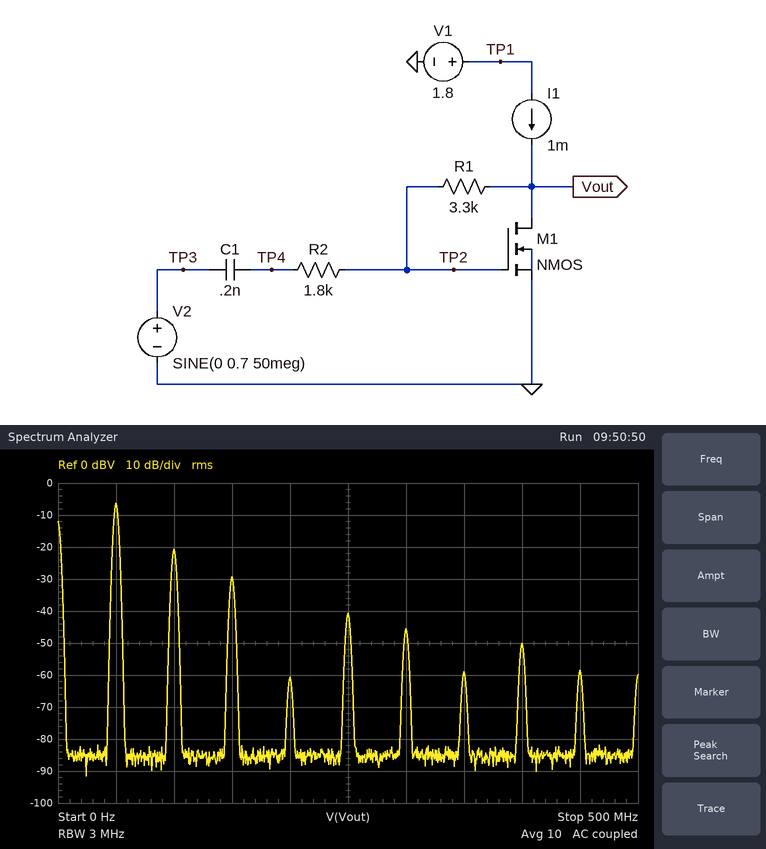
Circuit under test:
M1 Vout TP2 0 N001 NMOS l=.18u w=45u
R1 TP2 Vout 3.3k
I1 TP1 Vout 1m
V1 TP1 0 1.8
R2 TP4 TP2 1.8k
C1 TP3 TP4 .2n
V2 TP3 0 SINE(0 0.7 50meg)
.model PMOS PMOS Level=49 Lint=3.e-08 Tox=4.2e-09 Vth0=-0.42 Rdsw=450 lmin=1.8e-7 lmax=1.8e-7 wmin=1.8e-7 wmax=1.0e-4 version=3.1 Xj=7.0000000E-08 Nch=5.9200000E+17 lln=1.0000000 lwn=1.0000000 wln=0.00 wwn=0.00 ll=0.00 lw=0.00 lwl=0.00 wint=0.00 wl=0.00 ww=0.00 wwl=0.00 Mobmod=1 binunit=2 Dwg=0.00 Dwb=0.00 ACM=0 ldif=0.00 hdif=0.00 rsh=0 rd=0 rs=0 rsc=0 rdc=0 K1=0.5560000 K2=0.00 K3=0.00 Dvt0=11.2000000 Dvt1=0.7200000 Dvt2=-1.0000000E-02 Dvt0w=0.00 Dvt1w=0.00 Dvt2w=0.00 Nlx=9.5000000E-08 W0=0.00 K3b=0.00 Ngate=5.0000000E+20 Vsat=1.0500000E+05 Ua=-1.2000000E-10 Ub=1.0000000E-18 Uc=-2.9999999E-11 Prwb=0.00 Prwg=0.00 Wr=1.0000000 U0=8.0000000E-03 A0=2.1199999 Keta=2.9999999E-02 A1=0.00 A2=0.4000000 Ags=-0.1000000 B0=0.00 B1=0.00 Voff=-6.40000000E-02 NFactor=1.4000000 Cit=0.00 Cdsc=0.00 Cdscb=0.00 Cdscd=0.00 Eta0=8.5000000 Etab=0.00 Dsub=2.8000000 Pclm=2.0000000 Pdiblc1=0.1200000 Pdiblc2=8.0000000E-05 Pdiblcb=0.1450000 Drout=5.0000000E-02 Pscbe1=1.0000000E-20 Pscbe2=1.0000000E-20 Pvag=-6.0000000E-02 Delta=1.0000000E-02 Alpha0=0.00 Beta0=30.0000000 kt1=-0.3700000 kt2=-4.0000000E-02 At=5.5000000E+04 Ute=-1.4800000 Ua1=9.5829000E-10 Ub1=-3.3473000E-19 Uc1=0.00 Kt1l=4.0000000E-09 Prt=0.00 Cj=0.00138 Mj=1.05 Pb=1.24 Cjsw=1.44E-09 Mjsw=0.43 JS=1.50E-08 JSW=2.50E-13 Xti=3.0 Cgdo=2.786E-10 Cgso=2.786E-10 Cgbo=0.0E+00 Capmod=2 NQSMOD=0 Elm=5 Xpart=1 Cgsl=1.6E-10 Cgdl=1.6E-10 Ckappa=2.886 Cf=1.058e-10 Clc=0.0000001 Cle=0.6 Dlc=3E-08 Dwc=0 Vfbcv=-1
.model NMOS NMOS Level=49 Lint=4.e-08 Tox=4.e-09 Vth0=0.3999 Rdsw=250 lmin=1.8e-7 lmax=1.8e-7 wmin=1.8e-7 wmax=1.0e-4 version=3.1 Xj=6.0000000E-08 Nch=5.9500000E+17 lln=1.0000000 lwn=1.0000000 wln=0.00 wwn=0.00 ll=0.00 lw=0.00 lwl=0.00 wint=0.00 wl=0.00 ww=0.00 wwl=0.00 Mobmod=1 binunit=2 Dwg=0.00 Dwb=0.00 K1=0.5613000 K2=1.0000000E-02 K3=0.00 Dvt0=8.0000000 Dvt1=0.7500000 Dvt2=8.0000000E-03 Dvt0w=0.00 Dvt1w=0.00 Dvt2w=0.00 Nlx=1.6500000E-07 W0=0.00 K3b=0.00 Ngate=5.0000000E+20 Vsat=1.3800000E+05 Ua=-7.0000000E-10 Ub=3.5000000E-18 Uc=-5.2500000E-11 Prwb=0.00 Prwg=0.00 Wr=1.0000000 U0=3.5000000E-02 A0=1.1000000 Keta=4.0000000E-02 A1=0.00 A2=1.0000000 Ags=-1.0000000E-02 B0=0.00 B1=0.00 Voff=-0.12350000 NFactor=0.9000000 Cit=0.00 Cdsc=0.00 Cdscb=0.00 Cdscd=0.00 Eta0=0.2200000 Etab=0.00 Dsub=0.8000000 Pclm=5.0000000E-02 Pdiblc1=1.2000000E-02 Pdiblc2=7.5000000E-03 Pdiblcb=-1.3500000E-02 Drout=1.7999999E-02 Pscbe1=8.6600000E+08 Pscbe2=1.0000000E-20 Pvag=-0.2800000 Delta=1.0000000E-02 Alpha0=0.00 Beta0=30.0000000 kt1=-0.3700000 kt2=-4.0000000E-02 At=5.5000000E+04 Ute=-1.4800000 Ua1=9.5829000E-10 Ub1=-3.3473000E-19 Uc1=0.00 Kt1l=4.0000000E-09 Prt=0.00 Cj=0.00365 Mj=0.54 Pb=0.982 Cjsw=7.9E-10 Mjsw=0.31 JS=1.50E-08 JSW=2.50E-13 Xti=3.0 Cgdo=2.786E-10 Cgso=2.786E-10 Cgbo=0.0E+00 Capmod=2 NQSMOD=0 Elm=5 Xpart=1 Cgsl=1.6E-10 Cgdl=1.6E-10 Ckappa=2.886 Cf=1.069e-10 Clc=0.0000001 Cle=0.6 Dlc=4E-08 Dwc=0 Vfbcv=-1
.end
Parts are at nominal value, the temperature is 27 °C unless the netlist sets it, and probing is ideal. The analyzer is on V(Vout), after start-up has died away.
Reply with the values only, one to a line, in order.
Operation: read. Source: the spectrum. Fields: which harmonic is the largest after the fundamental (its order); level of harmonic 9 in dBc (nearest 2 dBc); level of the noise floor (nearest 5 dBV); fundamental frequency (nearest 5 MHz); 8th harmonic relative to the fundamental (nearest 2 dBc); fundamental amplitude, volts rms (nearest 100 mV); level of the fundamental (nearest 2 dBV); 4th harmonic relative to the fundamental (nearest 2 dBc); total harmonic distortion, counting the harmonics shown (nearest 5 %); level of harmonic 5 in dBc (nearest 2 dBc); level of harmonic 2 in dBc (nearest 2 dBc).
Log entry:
2
-52 dBc
-85 dBV
50 MHz
-44 dBc
500 mV
-6 dBV
-54 dBc
20 %
-34 dBc
-14 dBc
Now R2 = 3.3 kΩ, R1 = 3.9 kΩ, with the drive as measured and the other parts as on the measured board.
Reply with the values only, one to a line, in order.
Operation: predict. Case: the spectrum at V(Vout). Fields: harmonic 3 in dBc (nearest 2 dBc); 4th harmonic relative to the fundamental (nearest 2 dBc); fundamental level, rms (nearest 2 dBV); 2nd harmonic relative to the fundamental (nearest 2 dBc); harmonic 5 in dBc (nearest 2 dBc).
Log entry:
-26 dBc
-34 dBc
-8 dBV
-20 dBc
-54 dBc
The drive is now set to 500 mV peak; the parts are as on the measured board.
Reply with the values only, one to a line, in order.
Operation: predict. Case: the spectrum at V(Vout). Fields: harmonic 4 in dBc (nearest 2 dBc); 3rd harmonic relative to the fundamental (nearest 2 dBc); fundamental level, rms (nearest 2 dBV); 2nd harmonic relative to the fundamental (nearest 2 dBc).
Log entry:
-34 dBc
-26 dBc
-8 dBV
-20 dBc
